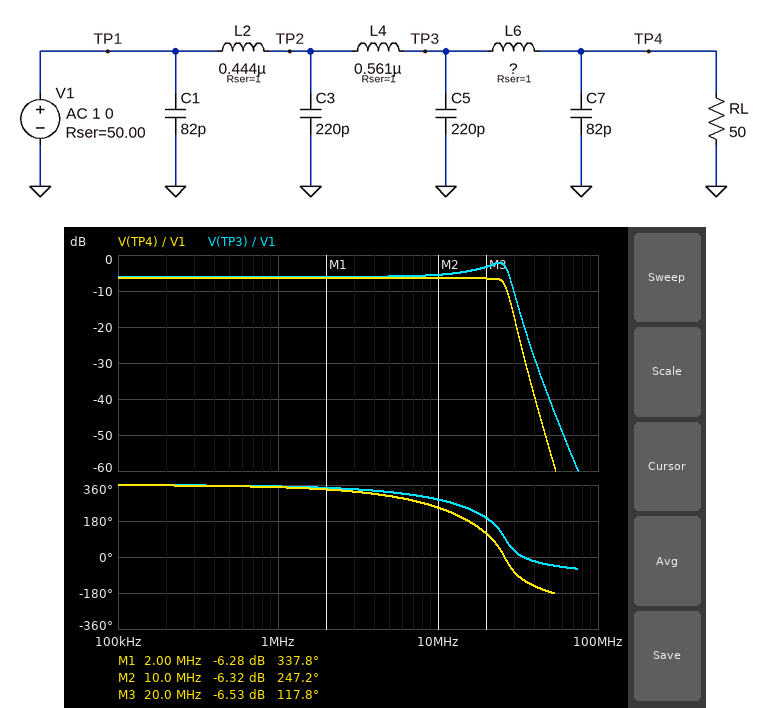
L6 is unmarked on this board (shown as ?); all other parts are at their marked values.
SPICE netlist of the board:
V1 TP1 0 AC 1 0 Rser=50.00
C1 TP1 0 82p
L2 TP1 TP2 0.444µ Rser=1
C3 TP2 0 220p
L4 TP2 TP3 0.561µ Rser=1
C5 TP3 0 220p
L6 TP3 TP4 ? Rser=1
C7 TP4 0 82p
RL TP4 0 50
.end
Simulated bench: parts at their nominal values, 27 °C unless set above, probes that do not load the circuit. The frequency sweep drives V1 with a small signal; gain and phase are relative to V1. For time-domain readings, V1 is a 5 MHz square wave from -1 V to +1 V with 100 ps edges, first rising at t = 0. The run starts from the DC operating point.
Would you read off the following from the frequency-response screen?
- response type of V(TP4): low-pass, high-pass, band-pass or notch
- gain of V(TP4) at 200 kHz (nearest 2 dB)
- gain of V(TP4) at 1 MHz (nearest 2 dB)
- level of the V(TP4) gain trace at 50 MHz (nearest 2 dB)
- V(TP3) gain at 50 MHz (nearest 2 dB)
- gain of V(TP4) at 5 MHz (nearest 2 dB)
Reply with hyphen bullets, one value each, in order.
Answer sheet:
- low-pass
- -6 dB
- -6 dB
- -54 dB
- -40 dB
- -6 dB
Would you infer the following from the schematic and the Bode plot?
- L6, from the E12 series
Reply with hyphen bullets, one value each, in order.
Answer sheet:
- 560 nH
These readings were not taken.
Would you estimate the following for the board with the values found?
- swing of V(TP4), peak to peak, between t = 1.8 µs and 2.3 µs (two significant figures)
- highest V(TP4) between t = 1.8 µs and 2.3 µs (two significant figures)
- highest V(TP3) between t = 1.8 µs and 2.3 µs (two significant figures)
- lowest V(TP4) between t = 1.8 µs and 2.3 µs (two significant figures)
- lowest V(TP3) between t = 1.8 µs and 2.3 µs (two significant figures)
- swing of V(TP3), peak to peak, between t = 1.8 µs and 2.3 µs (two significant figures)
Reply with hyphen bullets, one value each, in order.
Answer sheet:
- 1.3 V
- 660 mV
- 810 mV
- -660 mV
- -810 mV
- 1.6 V
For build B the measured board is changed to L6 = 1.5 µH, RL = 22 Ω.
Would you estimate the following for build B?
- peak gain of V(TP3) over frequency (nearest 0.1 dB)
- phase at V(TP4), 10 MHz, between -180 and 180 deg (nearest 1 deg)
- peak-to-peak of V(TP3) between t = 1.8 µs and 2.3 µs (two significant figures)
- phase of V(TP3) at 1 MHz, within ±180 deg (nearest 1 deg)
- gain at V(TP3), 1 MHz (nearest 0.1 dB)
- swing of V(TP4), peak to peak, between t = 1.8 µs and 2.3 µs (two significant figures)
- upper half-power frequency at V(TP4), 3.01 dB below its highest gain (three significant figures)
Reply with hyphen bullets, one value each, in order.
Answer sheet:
- -0.1 dB
- -148 deg
- 2.6 V
- 7 deg
- -9.7 dB
- 600 mV
- 9.60 MHz
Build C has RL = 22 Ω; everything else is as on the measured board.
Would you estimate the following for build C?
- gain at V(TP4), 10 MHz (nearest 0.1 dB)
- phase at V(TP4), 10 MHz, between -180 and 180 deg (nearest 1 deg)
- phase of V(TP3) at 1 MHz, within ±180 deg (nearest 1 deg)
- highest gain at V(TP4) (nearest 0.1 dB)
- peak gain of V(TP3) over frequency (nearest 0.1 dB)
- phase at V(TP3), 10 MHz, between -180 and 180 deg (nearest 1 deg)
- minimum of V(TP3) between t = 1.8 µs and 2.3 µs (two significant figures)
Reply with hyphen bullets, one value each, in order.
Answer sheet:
- -10.7 dB
- -114 deg
- -2 deg
- -10.6 dB
- 0.2 dB
- -52 deg
- -930 mV
